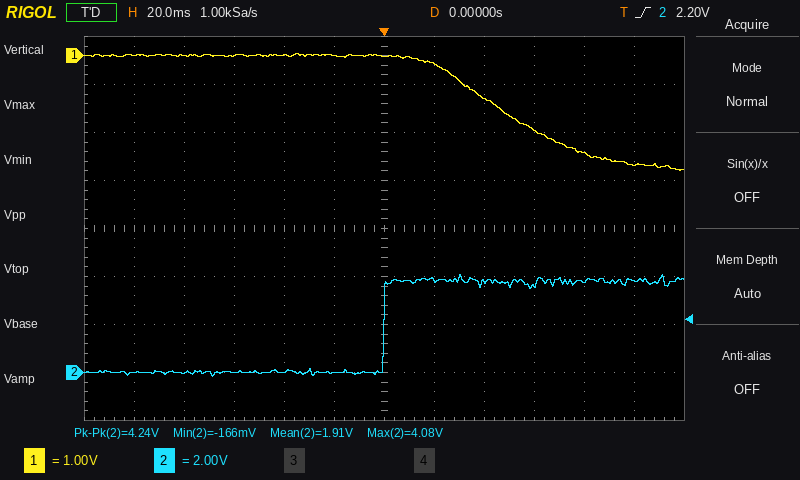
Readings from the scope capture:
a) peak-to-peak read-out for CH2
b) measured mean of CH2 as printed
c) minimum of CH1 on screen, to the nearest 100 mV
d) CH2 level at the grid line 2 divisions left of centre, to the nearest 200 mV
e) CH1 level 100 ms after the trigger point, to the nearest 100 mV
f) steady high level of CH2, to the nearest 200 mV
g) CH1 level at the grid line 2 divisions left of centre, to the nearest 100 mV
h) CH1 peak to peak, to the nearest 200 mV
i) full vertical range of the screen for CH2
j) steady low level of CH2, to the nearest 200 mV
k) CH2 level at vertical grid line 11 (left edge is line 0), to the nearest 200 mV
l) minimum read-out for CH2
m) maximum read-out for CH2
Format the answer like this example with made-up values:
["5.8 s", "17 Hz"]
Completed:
["4.24 V", "1.91 V", "-2.4 V", "0.0 V", "-2.3 V", "3.8 V", "0.0 V", "2.4 V", "16 V", "0.0 V", "3.8 V", "-166 mV", "4.08 V"]
